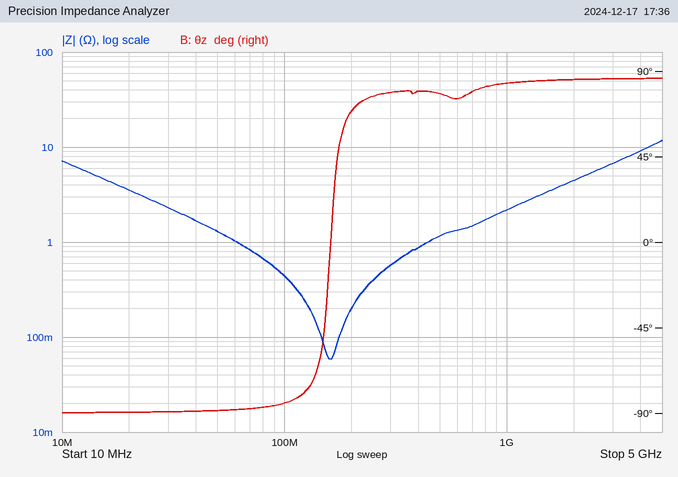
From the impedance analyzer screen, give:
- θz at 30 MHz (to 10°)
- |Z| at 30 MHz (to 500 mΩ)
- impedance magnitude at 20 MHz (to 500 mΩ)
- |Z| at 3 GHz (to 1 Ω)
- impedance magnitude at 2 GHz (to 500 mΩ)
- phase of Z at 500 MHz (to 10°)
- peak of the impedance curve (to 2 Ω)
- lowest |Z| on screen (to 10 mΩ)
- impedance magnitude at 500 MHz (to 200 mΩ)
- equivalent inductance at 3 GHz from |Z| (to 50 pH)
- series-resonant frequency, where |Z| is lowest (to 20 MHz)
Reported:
-90°
2.5 Ω
3.5 Ω
7 Ω
4.5 Ω
80°
12 Ω
60 mΩ
1.2 Ω
350 pH
160 MHz
